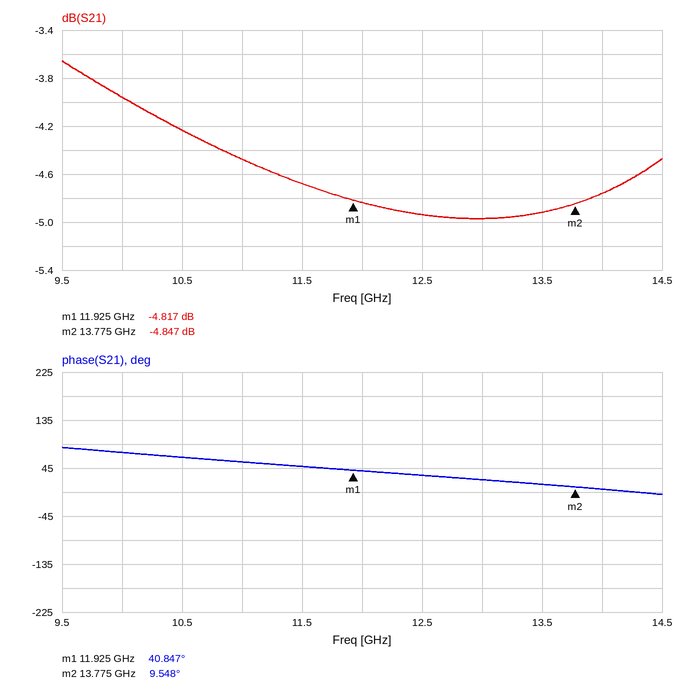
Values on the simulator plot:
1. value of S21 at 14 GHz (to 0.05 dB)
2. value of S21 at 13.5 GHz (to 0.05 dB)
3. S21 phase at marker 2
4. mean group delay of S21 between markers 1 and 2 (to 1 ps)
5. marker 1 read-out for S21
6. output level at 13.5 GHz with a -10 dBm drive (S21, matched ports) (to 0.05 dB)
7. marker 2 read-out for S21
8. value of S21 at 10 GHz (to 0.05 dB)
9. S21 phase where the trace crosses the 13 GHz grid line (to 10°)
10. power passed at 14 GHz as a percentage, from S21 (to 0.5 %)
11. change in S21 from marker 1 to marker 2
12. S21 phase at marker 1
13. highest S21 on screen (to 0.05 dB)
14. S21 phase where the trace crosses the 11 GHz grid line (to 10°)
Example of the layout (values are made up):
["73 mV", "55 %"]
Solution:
["-4.75 dB", "-4.90 dB", "9.548°", "47 ps", "-4.817 dB", "-14.90 dBm", "-4.847 dB", "-3.95 dB", "20°", "33.5 %", "-0.030 dB", "40.847°", "-3.65 dB", "60°"]
